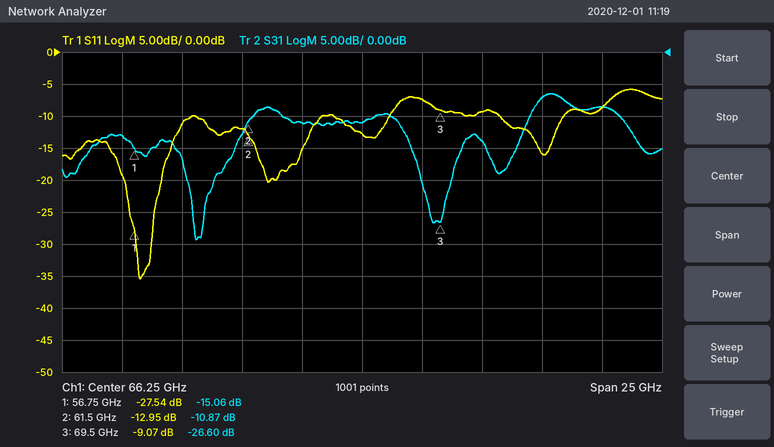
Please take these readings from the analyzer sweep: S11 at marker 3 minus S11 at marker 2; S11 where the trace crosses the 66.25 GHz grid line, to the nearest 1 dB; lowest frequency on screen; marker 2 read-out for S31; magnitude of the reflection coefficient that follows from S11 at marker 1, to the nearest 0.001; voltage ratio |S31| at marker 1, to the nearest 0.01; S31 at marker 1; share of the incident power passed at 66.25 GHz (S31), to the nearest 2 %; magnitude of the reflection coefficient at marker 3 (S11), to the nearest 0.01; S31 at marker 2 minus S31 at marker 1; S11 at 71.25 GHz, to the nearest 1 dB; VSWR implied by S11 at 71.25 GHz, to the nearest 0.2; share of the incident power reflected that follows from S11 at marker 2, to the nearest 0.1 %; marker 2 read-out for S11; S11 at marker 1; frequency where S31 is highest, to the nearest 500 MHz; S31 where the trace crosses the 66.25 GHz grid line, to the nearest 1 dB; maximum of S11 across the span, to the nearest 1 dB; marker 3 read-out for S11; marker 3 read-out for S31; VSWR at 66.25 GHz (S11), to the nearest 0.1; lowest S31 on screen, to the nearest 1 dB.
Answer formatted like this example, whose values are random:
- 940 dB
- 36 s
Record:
- 3.88 dB
- -13 dB
- 53.75 GHz
- -10.87 dB
- 0.042
- 0.18
- -15.06 dB
- 8 %
- 0.35
- 4.19 dB
- -9 dB
- 2.0
- 5.1 %
- -12.95 dB
- -27.54 dB
- 74.0 GHz
- -11 dB
- -6 dB
- -9.07 dB
- -26.60 dB
- 1.6
- -29 dB
